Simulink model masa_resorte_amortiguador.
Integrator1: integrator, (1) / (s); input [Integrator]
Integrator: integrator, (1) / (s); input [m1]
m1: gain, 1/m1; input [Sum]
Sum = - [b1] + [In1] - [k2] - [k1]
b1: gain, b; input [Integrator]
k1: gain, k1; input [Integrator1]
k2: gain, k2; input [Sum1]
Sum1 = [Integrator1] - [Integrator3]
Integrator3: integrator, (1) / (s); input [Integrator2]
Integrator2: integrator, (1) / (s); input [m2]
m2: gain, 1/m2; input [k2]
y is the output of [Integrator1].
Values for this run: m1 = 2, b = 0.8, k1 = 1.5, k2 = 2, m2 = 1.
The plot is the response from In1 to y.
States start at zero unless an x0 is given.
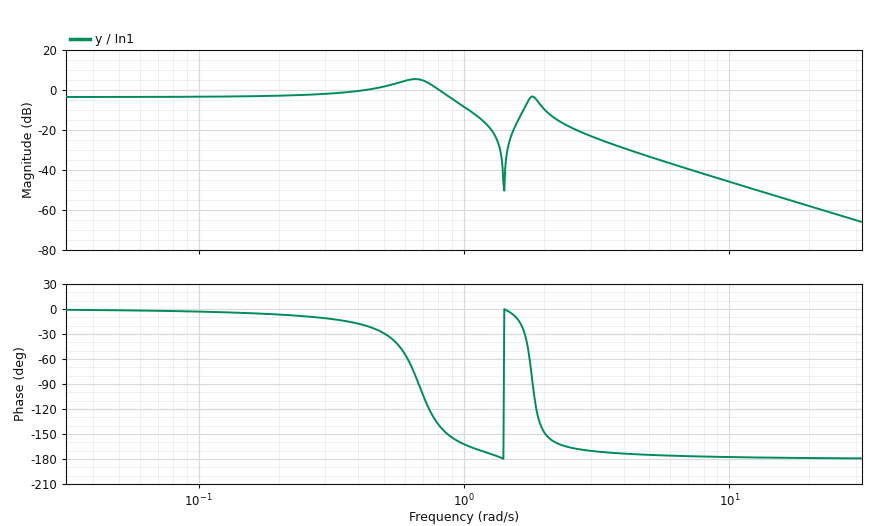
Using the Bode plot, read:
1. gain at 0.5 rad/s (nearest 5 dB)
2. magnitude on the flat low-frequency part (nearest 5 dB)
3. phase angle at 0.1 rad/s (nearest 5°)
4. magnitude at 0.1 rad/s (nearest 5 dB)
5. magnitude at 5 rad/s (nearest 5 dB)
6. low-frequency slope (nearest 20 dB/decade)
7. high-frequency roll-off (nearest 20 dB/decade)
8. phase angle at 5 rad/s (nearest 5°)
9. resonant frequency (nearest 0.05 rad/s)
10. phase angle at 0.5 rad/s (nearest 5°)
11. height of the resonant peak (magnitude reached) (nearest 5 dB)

0 dB
-5 dB
-5°
-5 dB
-35 dB
0 dB/decade
-40 dB/decade
-175°
0.65 rad/s
-30°
5 dB
